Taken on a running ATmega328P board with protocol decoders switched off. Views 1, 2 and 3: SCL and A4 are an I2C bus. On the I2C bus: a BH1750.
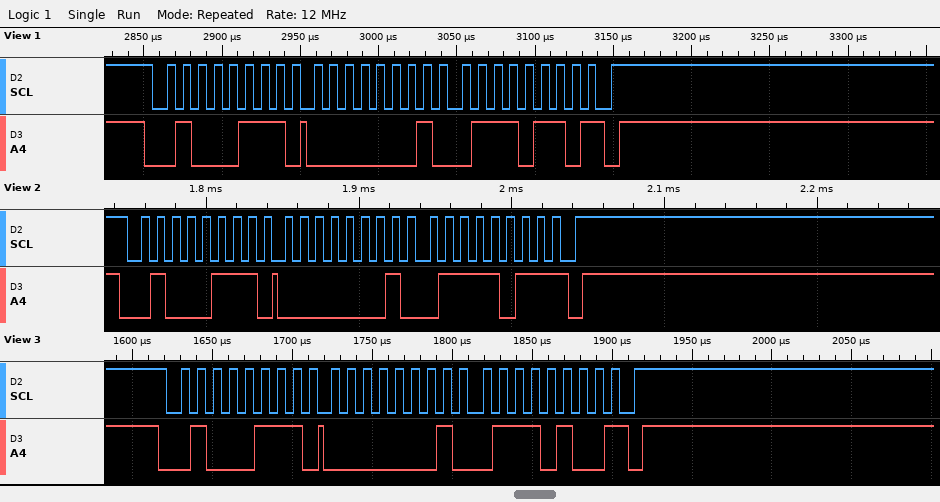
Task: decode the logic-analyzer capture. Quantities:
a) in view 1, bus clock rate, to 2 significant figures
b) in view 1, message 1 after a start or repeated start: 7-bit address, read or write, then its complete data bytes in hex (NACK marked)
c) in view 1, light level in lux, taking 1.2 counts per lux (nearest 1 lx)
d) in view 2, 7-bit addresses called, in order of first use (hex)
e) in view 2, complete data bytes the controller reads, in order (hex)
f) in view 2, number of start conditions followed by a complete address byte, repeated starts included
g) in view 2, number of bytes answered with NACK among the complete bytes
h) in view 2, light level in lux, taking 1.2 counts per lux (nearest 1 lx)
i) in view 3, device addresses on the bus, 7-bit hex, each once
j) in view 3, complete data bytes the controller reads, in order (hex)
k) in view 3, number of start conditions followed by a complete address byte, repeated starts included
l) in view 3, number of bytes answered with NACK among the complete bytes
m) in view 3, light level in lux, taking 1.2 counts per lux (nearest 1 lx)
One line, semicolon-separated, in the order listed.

100 kHz; 0x23 read: 01 76 NACK; 312 lx; 0x23; 01 7B; 1; 1; 316 lx; 0x23; 01 74; 1; 1; 310 lx
